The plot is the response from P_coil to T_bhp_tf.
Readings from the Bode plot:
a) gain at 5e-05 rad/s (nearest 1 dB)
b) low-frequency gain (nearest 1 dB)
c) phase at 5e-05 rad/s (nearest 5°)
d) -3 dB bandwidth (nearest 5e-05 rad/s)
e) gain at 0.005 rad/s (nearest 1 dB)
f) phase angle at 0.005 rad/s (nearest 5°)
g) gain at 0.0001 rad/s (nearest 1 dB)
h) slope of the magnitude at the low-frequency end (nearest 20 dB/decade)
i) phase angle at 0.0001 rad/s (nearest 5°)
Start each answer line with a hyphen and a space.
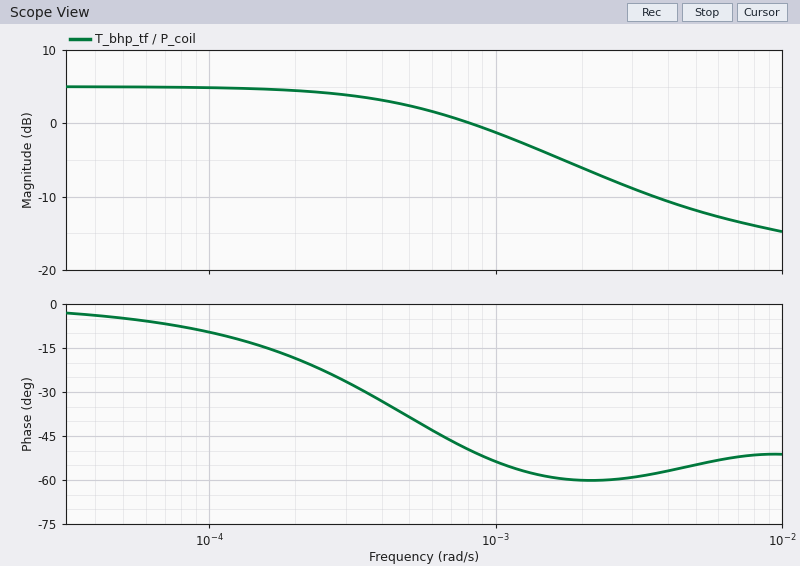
- 5 dB
- 5 dB
- -5°
- 0.00055 rad/s
- -12 dB
- -55°
- 5 dB
- 0 dB/decade
- -10°
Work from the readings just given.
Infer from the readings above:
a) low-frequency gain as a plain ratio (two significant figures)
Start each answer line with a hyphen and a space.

- 1.8
